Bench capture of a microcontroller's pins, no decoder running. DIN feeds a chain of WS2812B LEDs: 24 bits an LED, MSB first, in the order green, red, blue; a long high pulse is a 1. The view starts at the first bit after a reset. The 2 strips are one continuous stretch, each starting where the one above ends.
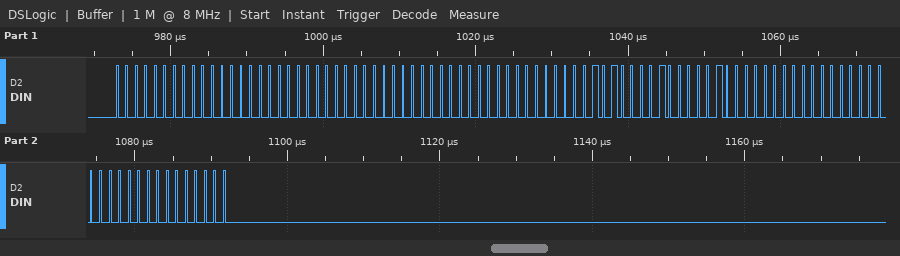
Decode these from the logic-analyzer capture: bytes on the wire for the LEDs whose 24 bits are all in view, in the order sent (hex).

00 00 00 00 00 00 28 41 00 00 00 00
